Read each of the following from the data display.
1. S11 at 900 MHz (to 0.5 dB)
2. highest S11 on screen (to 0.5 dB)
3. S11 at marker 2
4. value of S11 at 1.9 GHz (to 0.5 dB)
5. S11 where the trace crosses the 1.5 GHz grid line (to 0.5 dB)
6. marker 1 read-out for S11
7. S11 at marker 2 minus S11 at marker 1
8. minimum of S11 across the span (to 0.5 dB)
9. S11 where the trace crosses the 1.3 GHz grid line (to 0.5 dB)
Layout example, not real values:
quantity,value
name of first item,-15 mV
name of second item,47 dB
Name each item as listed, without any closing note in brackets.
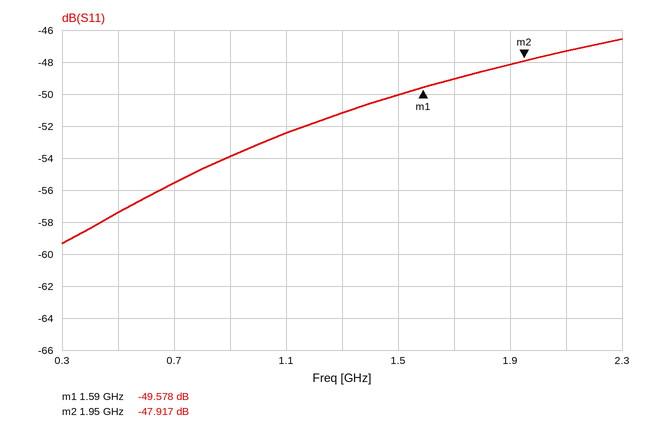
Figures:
quantity,value
S11 at 900 MHz,-54.0 dB
highest S11 on screen,-46.5 dB
S11 at marker 2,-47.917 dB
value of S11 at 1.9 GHz,-48.0 dB
S11 where the trace crosses the 1.5 GHz grid line,-50.0 dB
marker 1 read-out for S11,-49.578 dB
S11 at marker 2 minus S11 at marker 1,1.661 dB
minimum of S11 across the span,-59.5 dB
S11 where the trace crosses the 1.3 GHz grid line,-51.0 dB
